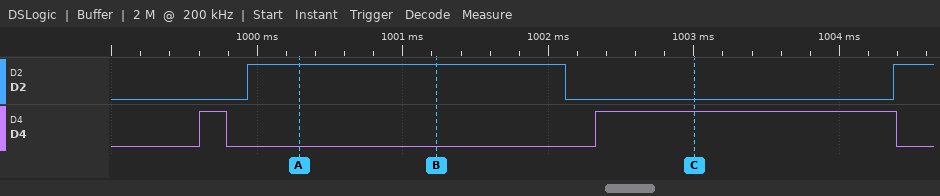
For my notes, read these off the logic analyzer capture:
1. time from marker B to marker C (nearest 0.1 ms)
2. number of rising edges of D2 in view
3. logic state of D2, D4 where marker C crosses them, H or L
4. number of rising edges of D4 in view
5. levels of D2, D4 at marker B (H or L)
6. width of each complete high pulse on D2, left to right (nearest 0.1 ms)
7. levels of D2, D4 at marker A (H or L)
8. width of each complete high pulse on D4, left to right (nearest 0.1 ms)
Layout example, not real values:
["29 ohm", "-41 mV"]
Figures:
["1.8 ms", "2", "D2=L, D4=H", "2", "D2=H, D4=L", "2.2 ms", "D2=H, D4=L", "0.2 ms, 2.1 ms"]
